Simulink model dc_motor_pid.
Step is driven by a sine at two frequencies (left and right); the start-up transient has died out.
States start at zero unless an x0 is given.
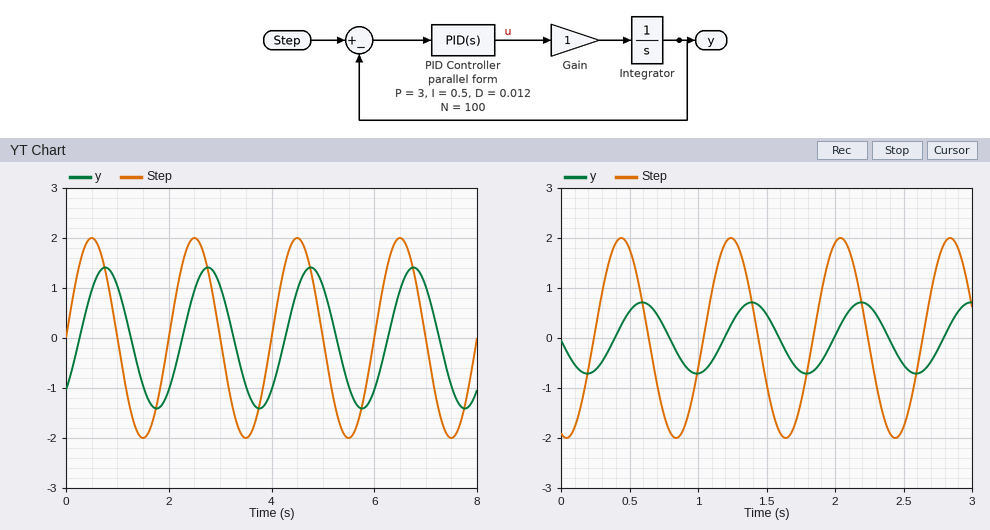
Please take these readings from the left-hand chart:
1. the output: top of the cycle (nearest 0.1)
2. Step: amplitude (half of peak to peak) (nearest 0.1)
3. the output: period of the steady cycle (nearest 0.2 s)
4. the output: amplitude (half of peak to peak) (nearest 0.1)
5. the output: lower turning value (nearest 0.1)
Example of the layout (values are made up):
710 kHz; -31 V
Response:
1.4; 2.0; 2.0 s; 1.4; -1.4
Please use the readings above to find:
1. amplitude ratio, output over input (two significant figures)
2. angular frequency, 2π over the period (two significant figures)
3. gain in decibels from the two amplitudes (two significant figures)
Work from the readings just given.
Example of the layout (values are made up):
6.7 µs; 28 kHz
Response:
0.70; 3.1 rad/s; -3.1 dB
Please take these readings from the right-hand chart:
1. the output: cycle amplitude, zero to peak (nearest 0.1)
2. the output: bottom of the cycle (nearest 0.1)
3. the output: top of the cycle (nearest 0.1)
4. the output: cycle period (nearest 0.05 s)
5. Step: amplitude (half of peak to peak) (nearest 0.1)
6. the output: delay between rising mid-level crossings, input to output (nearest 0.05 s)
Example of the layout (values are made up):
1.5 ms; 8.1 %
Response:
0.7; -0.7; 0.7; 0.80 s; 2.0; 0.15 s
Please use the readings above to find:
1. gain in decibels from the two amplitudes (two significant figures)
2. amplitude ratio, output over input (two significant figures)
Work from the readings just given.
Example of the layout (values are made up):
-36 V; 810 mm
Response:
-9.1 dB; 0.35
